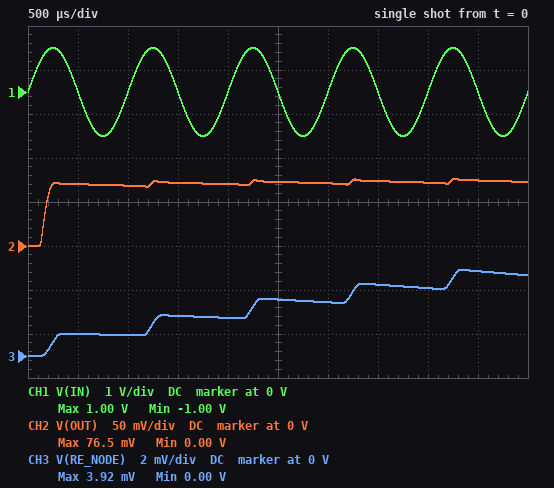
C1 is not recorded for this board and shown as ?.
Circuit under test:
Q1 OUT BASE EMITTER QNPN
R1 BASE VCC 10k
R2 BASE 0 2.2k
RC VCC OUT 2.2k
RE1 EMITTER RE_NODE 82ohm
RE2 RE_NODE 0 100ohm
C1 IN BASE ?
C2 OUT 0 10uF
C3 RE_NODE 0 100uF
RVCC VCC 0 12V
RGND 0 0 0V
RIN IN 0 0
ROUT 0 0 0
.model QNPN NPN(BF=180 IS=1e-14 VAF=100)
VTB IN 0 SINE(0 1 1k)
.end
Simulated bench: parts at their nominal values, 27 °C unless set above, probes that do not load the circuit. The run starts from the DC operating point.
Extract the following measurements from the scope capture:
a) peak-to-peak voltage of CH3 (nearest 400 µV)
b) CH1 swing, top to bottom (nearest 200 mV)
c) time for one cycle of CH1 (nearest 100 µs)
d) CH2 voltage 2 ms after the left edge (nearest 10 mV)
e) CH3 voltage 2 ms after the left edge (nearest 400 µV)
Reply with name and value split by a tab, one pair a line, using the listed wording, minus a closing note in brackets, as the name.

peak-to-peak voltage of CH3	4.0 mV
CH1 swing, top to bottom	2.0 V
time for one cycle of CH1	1.0 ms
CH2 voltage 2 ms after the left edge	70 mV
CH3 voltage 2 ms after the left edge	1.6 mV
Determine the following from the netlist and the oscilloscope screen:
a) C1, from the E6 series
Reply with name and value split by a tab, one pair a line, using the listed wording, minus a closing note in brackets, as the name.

C1, from the E6 series	3.3 µF
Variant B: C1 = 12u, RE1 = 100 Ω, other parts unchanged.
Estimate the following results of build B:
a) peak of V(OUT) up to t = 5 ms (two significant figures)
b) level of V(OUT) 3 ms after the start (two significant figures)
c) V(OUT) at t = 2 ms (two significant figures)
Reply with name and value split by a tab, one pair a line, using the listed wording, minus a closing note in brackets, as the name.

peak of V(OUT) up to t = 5 ms	160 mV
level of V(OUT) 3 ms after the start	140 mV
V(OUT) at t = 2 ms	150 mV
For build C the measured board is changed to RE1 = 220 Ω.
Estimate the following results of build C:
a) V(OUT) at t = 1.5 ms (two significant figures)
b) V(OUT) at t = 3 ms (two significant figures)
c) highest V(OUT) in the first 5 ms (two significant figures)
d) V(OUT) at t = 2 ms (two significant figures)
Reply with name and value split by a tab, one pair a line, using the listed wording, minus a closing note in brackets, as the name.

V(OUT) at t = 1.5 ms	80 mV
V(OUT) at t = 3 ms	82 mV
highest V(OUT) in the first 5 ms	92 mV
V(OUT) at t = 2 ms	78 mV
